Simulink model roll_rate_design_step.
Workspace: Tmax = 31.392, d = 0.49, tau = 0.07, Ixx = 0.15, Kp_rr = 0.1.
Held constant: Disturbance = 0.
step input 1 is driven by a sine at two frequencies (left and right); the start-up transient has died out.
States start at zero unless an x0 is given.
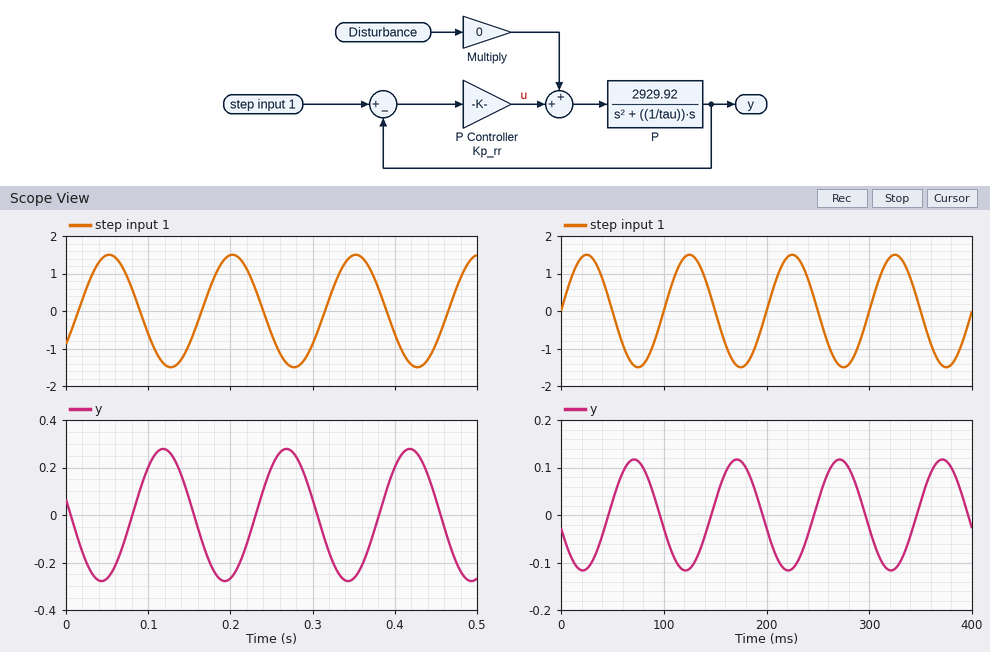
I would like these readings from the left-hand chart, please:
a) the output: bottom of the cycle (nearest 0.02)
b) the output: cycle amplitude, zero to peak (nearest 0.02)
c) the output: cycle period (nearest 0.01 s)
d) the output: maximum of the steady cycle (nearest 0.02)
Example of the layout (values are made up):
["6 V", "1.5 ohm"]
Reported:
["-0.28", "0.28", "0.15 s", "0.28"]
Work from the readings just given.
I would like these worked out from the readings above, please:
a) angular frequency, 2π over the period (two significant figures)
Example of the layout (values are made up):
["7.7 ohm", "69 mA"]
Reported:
["42 rad/s"]
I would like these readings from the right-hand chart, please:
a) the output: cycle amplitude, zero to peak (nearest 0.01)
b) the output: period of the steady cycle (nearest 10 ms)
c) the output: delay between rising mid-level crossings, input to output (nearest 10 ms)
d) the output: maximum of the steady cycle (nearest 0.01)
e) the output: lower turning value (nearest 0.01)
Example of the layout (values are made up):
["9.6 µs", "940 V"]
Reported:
["0.12", "100 ms", "50 ms", "0.12", "-0.12"]
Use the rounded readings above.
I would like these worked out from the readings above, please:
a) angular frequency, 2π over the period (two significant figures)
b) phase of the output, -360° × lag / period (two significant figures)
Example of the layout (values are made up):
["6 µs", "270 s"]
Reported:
["0.063 rad/ms", "-180°"]
